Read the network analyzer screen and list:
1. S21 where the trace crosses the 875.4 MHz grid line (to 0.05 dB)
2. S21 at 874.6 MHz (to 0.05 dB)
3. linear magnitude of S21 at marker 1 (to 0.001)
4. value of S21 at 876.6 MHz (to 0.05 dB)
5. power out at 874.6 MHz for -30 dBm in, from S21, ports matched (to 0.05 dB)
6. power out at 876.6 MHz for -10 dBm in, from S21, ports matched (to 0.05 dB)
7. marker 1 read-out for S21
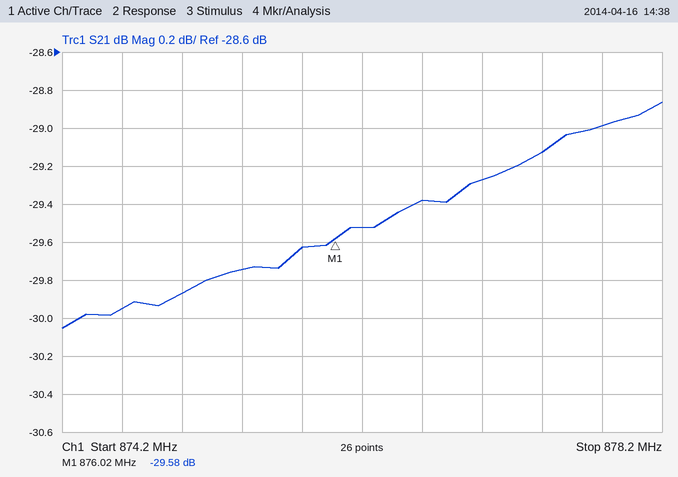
-29.75 dB
-29.95 dB
0.033
-29.40 dB
-59.95 dBm
-39.40 dBm
-29.58 dB
